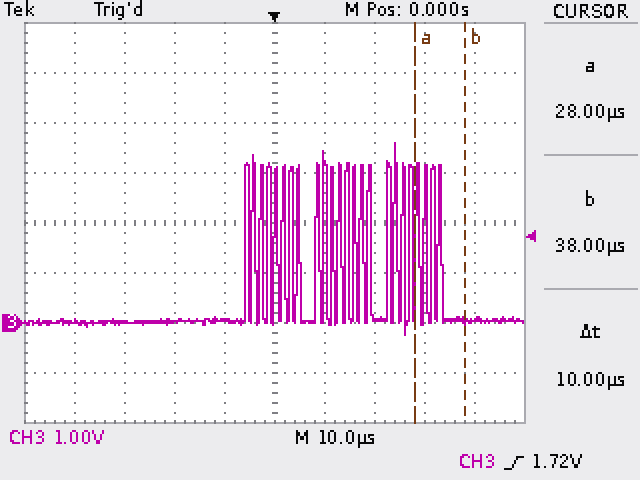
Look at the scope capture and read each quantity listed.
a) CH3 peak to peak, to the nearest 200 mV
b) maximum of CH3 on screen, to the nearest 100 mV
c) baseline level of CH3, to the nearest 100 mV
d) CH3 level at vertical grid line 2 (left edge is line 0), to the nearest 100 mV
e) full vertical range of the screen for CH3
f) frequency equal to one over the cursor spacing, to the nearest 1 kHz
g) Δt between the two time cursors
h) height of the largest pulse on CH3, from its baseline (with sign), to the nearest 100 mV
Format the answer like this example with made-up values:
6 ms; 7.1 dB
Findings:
3.8 V; 3.6 V; 0.0 V; 0.0 V; 8 V; 100 kHz; 10 µs; +3.6 V
